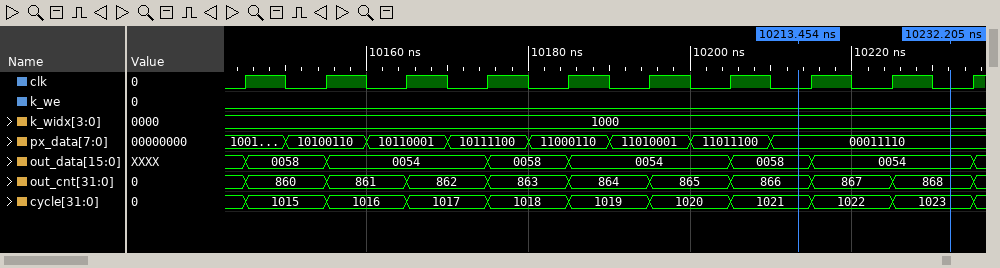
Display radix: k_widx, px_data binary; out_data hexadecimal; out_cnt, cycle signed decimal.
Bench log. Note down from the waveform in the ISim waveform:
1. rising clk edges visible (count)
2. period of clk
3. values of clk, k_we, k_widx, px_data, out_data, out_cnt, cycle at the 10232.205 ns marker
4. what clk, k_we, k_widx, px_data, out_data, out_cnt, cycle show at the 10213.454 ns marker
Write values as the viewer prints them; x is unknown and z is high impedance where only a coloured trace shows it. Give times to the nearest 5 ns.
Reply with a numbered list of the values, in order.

1. 10
2. 10 ns
3. clk=0, k_we=0, k_widx=1000, px_data=00011110, out_data=0054, out_cnt=868, cycle=1023
4. clk=0, k_we=0, k_widx=1000, px_data=00011110, out_data=0058, out_cnt=866, cycle=1021
